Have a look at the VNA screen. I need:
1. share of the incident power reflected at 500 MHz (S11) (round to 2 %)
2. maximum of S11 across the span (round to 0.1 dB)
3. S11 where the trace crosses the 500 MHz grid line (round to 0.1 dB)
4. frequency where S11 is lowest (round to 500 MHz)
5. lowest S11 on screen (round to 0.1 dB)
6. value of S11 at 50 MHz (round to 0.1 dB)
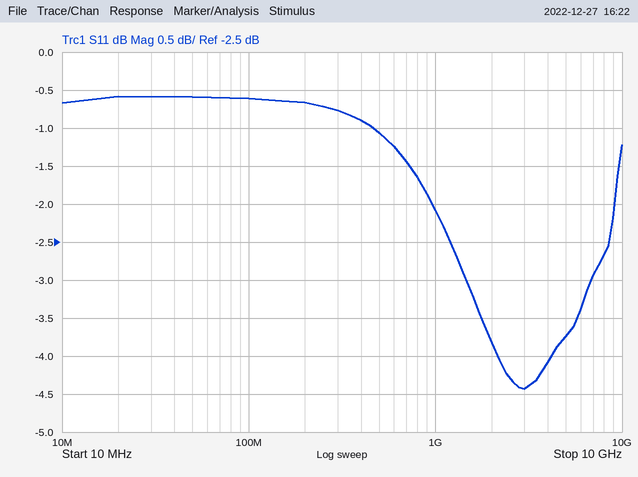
78 %
-0.6 dB
-1.1 dB
3.0 GHz
-4.4 dB
-0.6 dB
